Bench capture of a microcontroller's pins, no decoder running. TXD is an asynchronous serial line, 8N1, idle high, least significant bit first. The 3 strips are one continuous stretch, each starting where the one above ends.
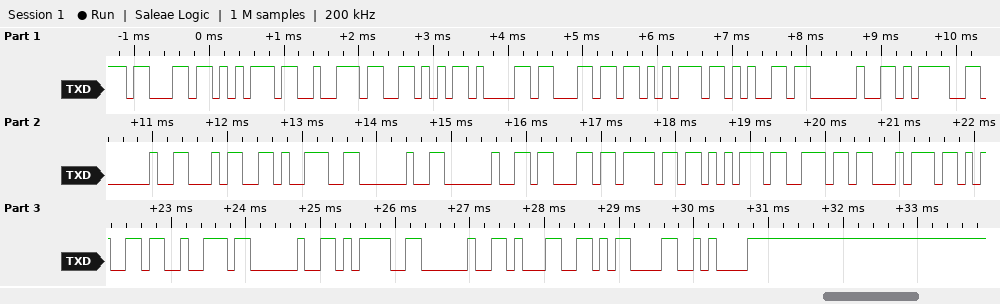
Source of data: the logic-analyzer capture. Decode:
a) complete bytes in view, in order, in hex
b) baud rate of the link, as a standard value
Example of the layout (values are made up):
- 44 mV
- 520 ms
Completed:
- 63 75 72 56 61 6C 75 65 20 3D 20 34 39 20 20 63 6F 75 6E 74 65 72 20 3D 20 31 0D 0A
- 9600 baud
